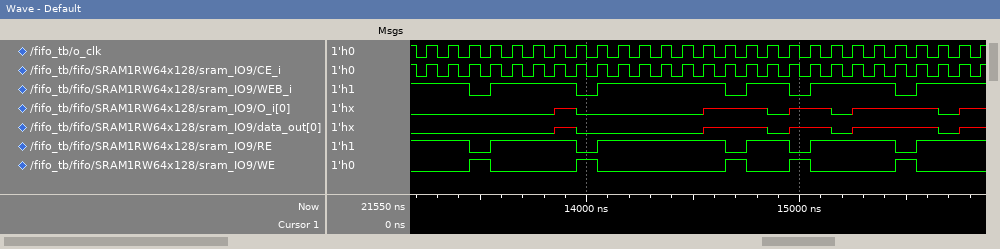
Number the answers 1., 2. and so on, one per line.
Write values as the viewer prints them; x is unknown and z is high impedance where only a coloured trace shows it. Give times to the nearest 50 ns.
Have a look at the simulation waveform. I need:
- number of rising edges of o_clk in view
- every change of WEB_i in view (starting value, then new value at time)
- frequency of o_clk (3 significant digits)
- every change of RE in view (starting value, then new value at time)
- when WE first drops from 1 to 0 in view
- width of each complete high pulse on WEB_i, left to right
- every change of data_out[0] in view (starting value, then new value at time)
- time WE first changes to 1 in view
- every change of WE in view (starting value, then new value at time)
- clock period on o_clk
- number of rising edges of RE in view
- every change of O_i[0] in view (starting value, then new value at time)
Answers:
1. 27
2. 1, 0 at 13450 ns, 1 at 13550 ns, 0 at 13950 ns, 1 at 14050 ns, 0 at 14650 ns, 1 at 14750 ns, 0 at 14950 ns, 1 at 15050 ns, 0 at 15450 ns, 1 at 15550 ns
3. 10.0 MHz
4. 1, 0 at 13450 ns, 1 at 13550 ns, 0 at 13950 ns, 1 at 14050 ns, 0 at 14650 ns, 1 at 14750 ns, 0 at 14950 ns, 1 at 15050 ns, 0 at 15450 ns, 1 at 15550 ns
5. 13550 ns
6. 400 ns, 600 ns, 200 ns, 400 ns
7. 0, x at 13850 ns, 0 at 13950 ns, x at 14550 ns, 0 at 14850 ns, x at 14950 ns, 0 at 15150 ns, x at 15250 ns, 0 at 15650 ns, x at 15750 ns
8. 13450 ns
9. 0, 1 at 13450 ns, 0 at 13550 ns, 1 at 13950 ns, 0 at 14050 ns, 1 at 14650 ns, 0 at 14750 ns, 1 at 14950 ns, 0 at 15050 ns, 1 at 15450 ns, 0 at 15550 ns
10. 100 ns
11. 5
12. 0, x at 13850 ns, 0 at 13950 ns, x at 14550 ns, 0 at 14850 ns, x at 14950 ns, 0 at 15150 ns, x at 15250 ns, 0 at 15650 ns, x at 15750 ns
